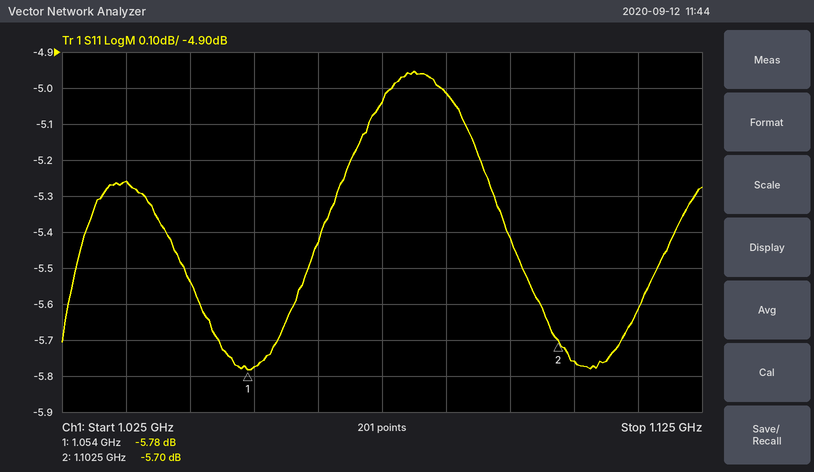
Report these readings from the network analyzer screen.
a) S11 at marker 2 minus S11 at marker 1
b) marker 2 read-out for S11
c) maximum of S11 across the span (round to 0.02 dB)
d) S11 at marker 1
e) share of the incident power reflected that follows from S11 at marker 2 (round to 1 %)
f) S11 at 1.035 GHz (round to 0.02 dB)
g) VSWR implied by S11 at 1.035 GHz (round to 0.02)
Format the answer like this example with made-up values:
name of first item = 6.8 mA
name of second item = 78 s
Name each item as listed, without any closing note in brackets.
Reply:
S11 at marker 2 minus S11 at marker 1 = 0.08 dB
marker 2 read-out for S11 = -5.70 dB
maximum of S11 across the span = -4.96 dB
S11 at marker 1 = -5.78 dB
share of the incident power reflected that follows from S11 at marker 2 = 27 %
S11 at 1.035 GHz = -5.26 dB
VSWR implied by S11 at 1.035 GHz = 3.40
